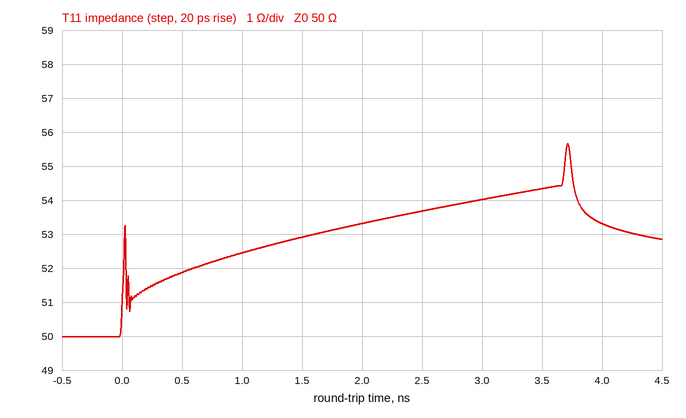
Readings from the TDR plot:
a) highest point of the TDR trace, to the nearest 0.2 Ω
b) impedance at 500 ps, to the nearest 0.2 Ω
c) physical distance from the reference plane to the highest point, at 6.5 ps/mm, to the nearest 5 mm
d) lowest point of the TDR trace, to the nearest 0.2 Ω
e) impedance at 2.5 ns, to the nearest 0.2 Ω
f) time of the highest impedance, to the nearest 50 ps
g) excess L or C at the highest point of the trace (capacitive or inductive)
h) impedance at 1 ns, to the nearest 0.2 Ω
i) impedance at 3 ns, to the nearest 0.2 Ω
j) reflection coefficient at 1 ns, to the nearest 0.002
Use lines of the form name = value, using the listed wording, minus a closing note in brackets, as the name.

highest point of the TDR trace, to the nearest 0.2 Ω = 55.6 Ω
impedance at 500 ps, to the nearest 0.2 Ω = 51.8 Ω
physical distance from the reference plane to the highest point, at 6.5 ps/mm, to the nearest 5 mm = 285 mm
lowest point of the TDR trace, to the nearest 0.2 Ω = 50.0 Ω
impedance at 2.5 ns, to the nearest 0.2 Ω = 53.6 Ω
time of the highest impedance, to the nearest 50 ps = 3.70 ns
excess L or C at the highest point of the trace = inductive
impedance at 1 ns, to the nearest 0.2 Ω = 52.4 Ω
impedance at 3 ns, to the nearest 0.2 Ω = 54.0 Ω
reflection coefficient at 1 ns, to the nearest 0.002 = +0.024
